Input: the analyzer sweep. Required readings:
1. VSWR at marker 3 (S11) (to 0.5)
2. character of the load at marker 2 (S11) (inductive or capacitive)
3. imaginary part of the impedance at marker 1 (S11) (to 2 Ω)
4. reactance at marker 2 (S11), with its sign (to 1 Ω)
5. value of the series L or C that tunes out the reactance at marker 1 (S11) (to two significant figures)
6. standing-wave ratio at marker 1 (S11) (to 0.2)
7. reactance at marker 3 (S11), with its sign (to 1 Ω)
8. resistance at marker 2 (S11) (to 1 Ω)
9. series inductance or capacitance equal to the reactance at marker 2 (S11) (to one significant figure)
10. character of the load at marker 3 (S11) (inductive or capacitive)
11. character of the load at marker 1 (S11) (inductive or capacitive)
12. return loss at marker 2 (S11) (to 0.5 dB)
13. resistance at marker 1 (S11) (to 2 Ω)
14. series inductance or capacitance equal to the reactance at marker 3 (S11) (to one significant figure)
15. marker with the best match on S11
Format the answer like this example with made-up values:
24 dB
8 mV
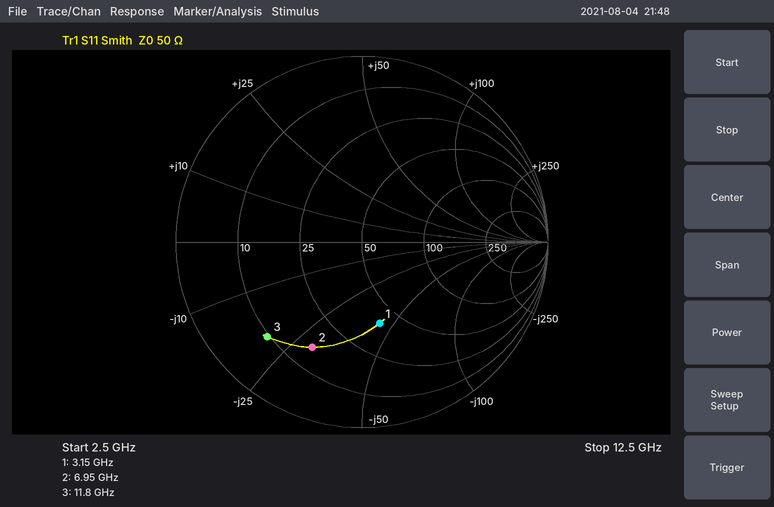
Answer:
6.0
capacitive
-44 Ω
-29 Ω
2.2 nH
2.6
-20 Ω
16 Ω
800 fF
capacitive
capacitive
4.0 dB
40 Ω
700 fF
marker 1
